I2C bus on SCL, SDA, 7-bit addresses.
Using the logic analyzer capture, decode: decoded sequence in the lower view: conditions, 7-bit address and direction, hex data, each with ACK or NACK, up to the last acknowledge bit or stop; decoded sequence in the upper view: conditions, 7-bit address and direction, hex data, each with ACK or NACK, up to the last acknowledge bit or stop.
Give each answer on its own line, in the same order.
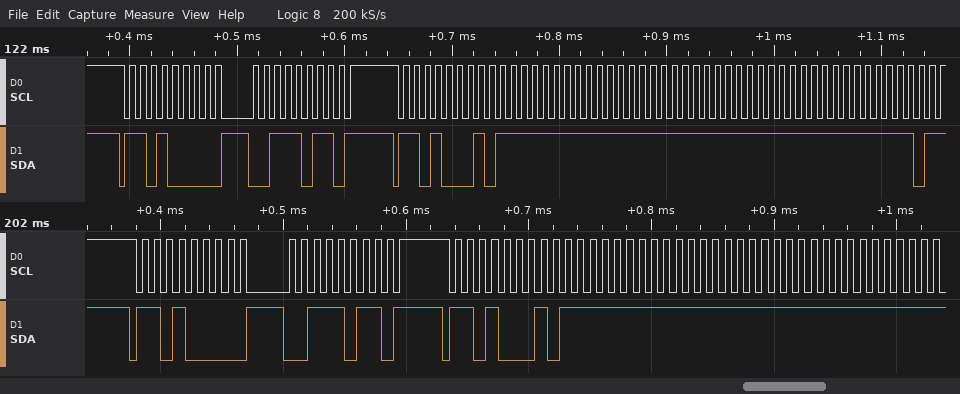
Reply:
start, address 68 write ACK, 3B ACK, repeated start, address 68 read ACK, FF NACK, FF NACK, FF NACK
start, address 68 write ACK, 3B ACK, repeated start, address 68 read ACK, FF NACK, FF NACK, FF NACK, FF NACK
